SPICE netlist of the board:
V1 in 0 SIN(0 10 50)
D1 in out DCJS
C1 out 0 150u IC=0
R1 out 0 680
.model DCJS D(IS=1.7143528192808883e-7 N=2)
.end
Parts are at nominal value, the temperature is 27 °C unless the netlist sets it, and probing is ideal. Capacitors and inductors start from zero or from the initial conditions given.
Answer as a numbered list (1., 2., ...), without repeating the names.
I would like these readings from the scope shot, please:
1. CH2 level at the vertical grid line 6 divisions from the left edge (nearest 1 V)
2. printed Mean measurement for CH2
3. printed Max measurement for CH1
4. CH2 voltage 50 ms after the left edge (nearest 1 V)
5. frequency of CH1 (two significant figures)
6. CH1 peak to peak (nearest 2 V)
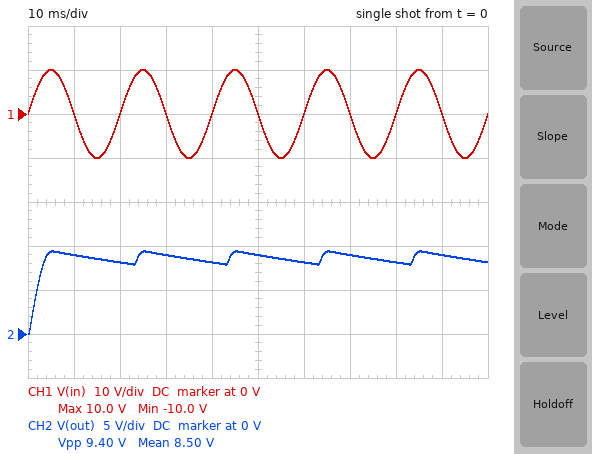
1. 8 V
2. 8.50 V
3. 10.0 V
4. 9 V
5. 50 Hz
6. 20 V
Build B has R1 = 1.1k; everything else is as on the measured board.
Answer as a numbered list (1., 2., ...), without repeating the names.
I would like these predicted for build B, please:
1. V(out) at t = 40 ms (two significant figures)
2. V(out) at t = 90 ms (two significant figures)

1. 8.6 V
2. 9.1 V
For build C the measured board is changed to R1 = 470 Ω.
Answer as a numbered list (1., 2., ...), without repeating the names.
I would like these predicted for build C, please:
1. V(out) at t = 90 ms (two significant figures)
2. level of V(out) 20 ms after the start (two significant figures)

1. 8.8 V
2. 7.6 V
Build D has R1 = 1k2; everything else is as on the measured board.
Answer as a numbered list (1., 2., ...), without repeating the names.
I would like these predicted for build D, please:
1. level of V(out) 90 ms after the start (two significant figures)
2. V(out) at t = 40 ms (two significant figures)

1. 9.2 V
2. 8.7 V
